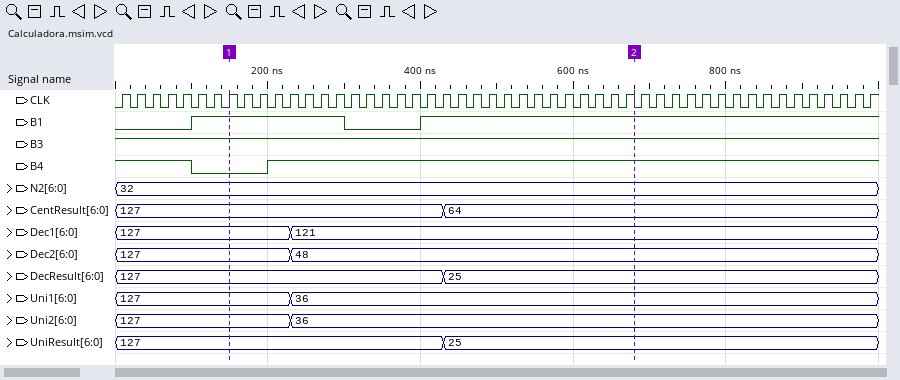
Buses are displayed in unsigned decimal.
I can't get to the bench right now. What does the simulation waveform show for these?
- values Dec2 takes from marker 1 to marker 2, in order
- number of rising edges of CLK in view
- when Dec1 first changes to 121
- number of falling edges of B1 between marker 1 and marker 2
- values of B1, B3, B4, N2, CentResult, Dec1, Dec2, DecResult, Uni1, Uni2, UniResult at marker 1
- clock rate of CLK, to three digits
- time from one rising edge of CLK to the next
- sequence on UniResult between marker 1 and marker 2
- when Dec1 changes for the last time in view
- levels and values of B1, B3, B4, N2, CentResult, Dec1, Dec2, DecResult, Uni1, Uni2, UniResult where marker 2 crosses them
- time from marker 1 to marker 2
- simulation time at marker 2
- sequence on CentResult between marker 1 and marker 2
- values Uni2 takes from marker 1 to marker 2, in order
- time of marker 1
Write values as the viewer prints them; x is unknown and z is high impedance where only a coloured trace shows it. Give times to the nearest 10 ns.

127, 48
50
230 ns
1
B1=1, B3=1, B4=0, N2=32, CentResult=127, Dec1=127, Dec2=127, DecResult=127, Uni1=127, Uni2=127, UniResult=127
50.0 MHz
20 ns
127, 25
230 ns
B1=1, B3=1, B4=1, N2=32, CentResult=64, Dec1=121, Dec2=48, DecResult=25, Uni1=36, Uni2=36, UniResult=25
530 ns
680 ns
127, 64
127, 36
150 ns
